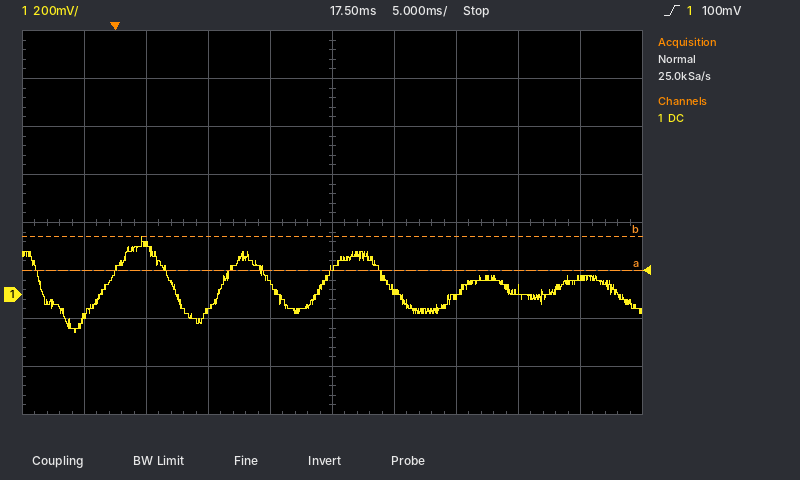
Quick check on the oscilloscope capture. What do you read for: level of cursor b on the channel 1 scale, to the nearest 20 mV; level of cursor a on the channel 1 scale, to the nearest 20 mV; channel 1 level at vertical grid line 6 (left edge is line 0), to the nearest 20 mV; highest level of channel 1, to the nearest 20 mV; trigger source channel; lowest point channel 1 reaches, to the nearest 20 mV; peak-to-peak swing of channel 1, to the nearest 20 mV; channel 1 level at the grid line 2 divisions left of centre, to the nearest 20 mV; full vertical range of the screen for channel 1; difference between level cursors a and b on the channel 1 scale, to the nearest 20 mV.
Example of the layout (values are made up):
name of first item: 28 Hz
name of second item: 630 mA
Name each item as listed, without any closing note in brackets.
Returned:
level of cursor b on the channel 1 scale, to the nearest 20 mV: 240 mV
level of cursor a on the channel 1 scale, to the nearest 20 mV: 100 mV
channel 1 level at vertical grid line 6 (left edge is line 0), to the nearest 20 mV: 20 mV
highest level of channel 1, to the nearest 20 mV: 240 mV
trigger source channel: channel 1
lowest point channel 1 reaches, to the nearest 20 mV: -160 mV
peak-to-peak swing of channel 1, to the nearest 20 mV: 400 mV
channel 1 level at the grid line 2 divisions left of centre, to the nearest 20 mV: -60 mV
full vertical range of the screen for channel 1: 1.6 V
difference between level cursors a and b on the channel 1 scale, to the nearest 20 mV: 140 mV
